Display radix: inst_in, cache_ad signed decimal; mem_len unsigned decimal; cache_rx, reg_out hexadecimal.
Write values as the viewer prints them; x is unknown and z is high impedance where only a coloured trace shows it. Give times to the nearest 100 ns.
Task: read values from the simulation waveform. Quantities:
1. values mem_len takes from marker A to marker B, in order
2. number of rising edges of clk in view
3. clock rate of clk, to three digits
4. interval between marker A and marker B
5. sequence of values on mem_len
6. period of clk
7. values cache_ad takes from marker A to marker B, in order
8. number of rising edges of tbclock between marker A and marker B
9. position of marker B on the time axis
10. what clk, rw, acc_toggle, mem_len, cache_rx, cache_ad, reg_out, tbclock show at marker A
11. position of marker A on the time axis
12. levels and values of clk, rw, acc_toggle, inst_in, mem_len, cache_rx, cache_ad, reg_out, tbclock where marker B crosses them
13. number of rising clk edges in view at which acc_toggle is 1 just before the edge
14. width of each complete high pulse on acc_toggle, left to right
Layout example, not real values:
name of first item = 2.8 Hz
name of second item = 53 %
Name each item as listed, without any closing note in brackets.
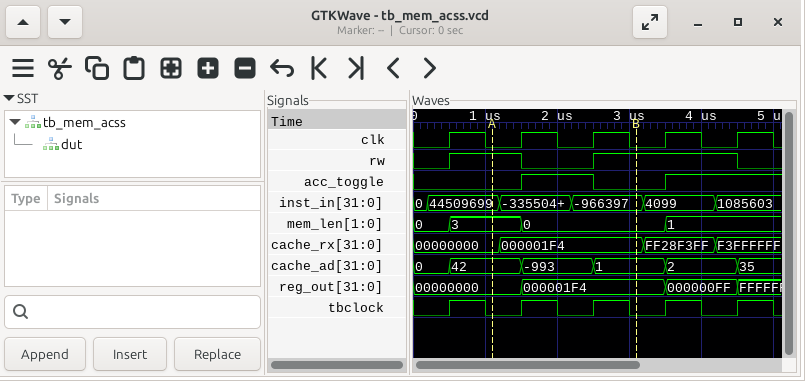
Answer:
values mem_len takes from marker A to marker B, in order = 3, 0
number of rising edges of clk in view = 5
clock rate of clk, to three digits = 1.00 MHz
interval between marker A and marker B = 2000 ns
sequence of values on mem_len = 0, 3, 0, 1
period of clk = 1000 ns
values cache_ad takes from marker A to marker B, in order = 42, -993, 1
number of rising edges of tbclock between marker A and marker B = 2
position of marker B on the time axis = 3100 ns
what clk, rw, acc_toggle, mem_len, cache_rx, cache_ad, reg_out, tbclock show at marker A = clk=0, rw=1, acc_toggle=0, mem_len=3, cache_rx=00000000, cache_ad=42, reg_out=00000000, tbclock=0
position of marker A on the time axis = 1100 ns
levels and values of clk, rw, acc_toggle, inst_in, mem_len, cache_rx, cache_ad, reg_out, tbclock where marker B crosses them = clk=0, rw=1, acc_toggle=0, inst_in=-966397, mem_len=0, cache_rx=000001F4, cache_ad=1, reg_out=000001F4, tbclock=0
number of rising clk edges in view at which acc_toggle is 1 just before the edge = 2
width of each complete high pulse on acc_toggle, left to right = 1000 ns
